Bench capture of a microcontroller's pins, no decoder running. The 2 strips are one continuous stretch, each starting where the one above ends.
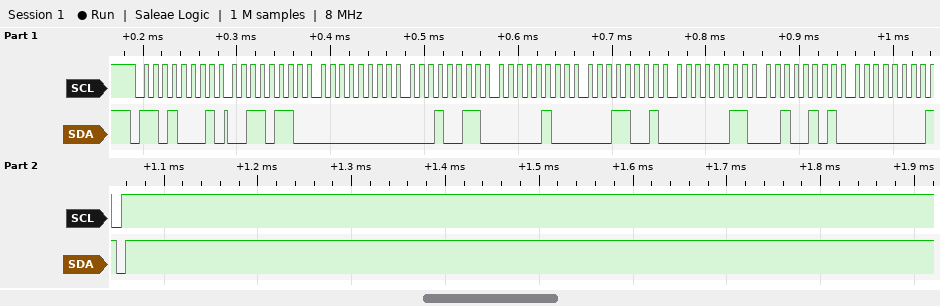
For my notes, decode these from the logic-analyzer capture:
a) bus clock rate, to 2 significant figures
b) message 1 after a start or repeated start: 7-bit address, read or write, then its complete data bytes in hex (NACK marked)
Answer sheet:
100 kHz
0x68 read: 36 00 13 04 19 03 25 00 NACK
